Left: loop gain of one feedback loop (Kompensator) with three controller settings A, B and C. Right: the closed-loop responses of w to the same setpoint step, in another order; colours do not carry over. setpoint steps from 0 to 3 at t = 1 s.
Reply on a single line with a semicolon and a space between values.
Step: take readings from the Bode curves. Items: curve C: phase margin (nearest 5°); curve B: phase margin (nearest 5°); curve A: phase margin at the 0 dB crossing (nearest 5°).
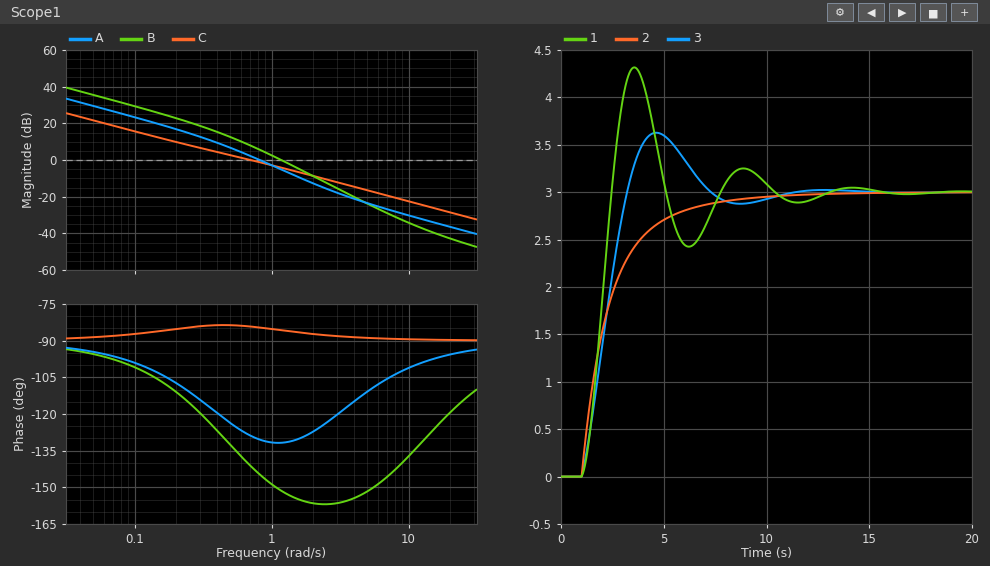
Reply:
95°; 30°; 50°
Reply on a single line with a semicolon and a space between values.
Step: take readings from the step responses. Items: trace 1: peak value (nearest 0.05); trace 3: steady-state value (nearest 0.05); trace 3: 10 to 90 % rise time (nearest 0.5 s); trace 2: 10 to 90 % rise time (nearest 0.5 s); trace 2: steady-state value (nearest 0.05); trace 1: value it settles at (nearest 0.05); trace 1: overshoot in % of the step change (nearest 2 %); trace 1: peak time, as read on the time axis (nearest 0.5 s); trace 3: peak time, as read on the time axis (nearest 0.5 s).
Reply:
4.30; 3.00; 1.5 s; 4.0 s; 3.00; 3.00; 44 %; 3.5 s; 4.5 s
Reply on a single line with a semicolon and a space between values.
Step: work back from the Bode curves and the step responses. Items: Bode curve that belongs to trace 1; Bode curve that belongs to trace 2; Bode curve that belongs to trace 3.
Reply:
B; C; A
